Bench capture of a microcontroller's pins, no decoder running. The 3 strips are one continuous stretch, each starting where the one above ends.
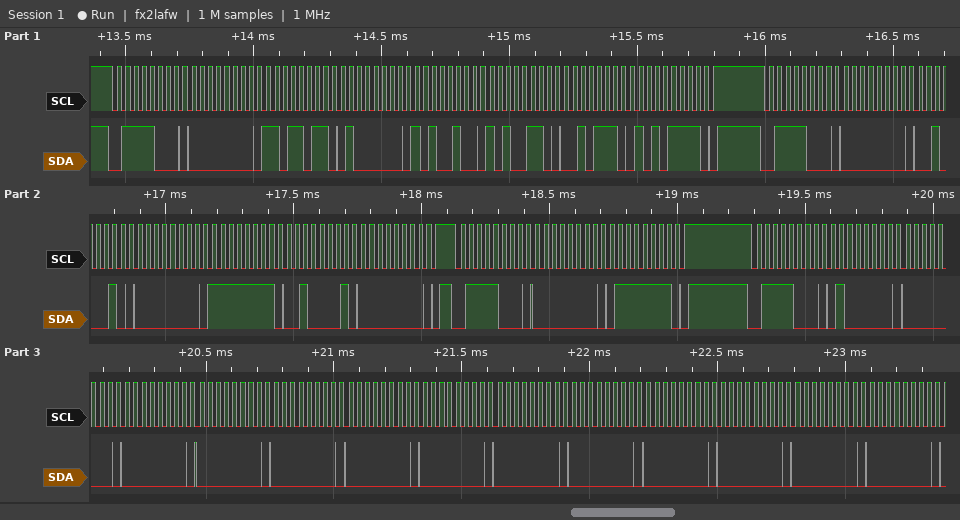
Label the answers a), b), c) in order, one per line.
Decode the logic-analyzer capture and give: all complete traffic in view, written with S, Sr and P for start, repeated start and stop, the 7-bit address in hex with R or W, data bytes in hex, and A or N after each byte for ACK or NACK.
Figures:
a) S 3CW A 00 A DB A 40 A A4 A A6 A 2E A AF A P S 3CW A 00 A 22 A 00 A FF A 21 A 00 A P S 3CW A 00 A 7F A P S 3CW A 40 A 00 A 00 A 00 A 00 A 00 A 00 A 00 A 00 A 00 A 00 A 00 A 00 A
